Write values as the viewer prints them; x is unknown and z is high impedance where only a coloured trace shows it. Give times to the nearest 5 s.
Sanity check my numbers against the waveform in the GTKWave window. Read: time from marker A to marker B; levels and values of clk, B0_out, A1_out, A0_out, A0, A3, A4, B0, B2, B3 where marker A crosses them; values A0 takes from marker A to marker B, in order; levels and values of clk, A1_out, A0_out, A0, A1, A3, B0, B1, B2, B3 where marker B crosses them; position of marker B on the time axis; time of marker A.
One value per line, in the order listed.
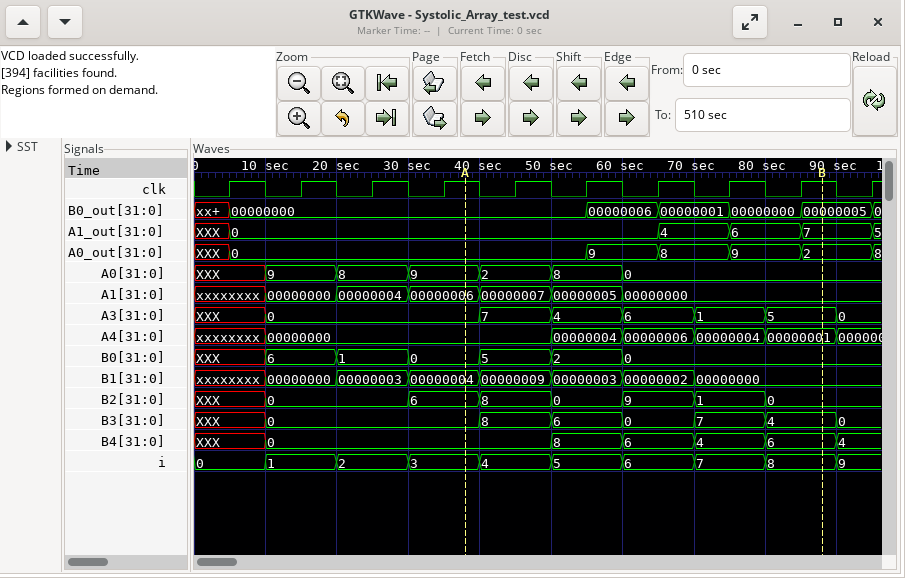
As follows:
50 s
clk=1, B0_out=00000000, A1_out=0, A0_out=0, A0=9, A3=0, A4=00000000, B0=0, B2=6, B3=0
9, 2, 8, 0
clk=1, A1_out=7, A0_out=2, A0=0, A1=00000000, A3=5, B0=0, B1=00000000, B2=0, B3=4
90 s
40 s
